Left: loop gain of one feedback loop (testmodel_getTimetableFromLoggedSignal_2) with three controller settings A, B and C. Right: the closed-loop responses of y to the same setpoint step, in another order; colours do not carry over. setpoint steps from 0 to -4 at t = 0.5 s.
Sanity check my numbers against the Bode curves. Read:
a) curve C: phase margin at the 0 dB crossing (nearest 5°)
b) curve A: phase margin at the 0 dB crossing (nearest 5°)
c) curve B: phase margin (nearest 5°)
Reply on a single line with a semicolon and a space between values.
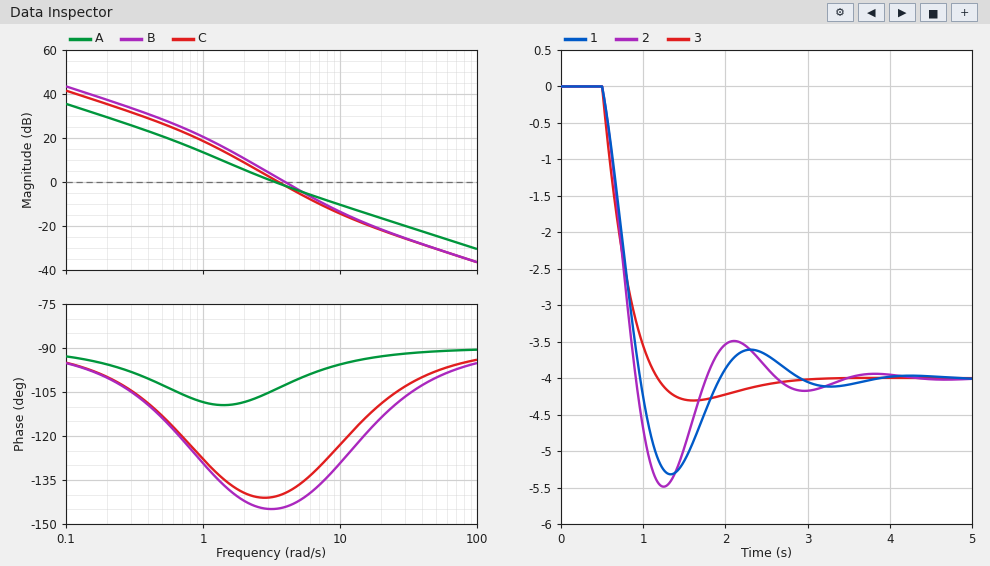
40°; 75°; 35°
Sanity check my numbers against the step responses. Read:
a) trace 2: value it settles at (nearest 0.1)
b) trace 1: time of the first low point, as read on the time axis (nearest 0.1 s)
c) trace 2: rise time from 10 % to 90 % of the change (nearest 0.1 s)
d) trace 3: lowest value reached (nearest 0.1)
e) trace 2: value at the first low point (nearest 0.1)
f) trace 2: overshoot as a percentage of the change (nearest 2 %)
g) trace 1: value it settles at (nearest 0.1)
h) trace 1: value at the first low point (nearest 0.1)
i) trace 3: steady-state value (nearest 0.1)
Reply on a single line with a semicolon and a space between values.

-4.0; 1.3 s; 0.3 s; -4.3; -5.5; 38 %; -4.0; -5.3; -4.0
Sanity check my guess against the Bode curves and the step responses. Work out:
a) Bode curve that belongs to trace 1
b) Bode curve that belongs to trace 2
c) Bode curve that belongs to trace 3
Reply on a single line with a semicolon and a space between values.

C; B; A
